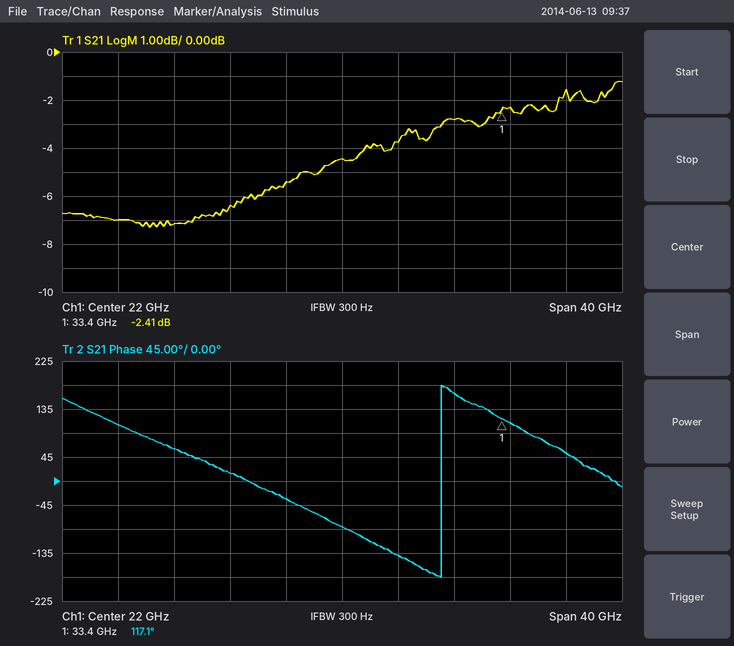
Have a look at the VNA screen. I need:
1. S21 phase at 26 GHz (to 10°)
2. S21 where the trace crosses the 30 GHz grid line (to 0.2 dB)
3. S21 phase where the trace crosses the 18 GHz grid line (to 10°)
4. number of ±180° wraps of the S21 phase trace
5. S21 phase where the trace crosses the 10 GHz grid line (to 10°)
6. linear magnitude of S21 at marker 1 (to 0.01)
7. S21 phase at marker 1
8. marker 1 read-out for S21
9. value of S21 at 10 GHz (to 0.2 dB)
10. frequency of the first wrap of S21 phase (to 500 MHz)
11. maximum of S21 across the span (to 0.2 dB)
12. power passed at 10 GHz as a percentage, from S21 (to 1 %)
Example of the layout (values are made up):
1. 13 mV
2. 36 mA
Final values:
1. -140°
2. -2.8 dB
3. -30°
4. 1
5. 60°
6. 0.76
7. 117.1°
8. -2.41 dB
9. -7.2 dB
10. 29.0 GHz
11. -1.2 dB
12. 19 %
